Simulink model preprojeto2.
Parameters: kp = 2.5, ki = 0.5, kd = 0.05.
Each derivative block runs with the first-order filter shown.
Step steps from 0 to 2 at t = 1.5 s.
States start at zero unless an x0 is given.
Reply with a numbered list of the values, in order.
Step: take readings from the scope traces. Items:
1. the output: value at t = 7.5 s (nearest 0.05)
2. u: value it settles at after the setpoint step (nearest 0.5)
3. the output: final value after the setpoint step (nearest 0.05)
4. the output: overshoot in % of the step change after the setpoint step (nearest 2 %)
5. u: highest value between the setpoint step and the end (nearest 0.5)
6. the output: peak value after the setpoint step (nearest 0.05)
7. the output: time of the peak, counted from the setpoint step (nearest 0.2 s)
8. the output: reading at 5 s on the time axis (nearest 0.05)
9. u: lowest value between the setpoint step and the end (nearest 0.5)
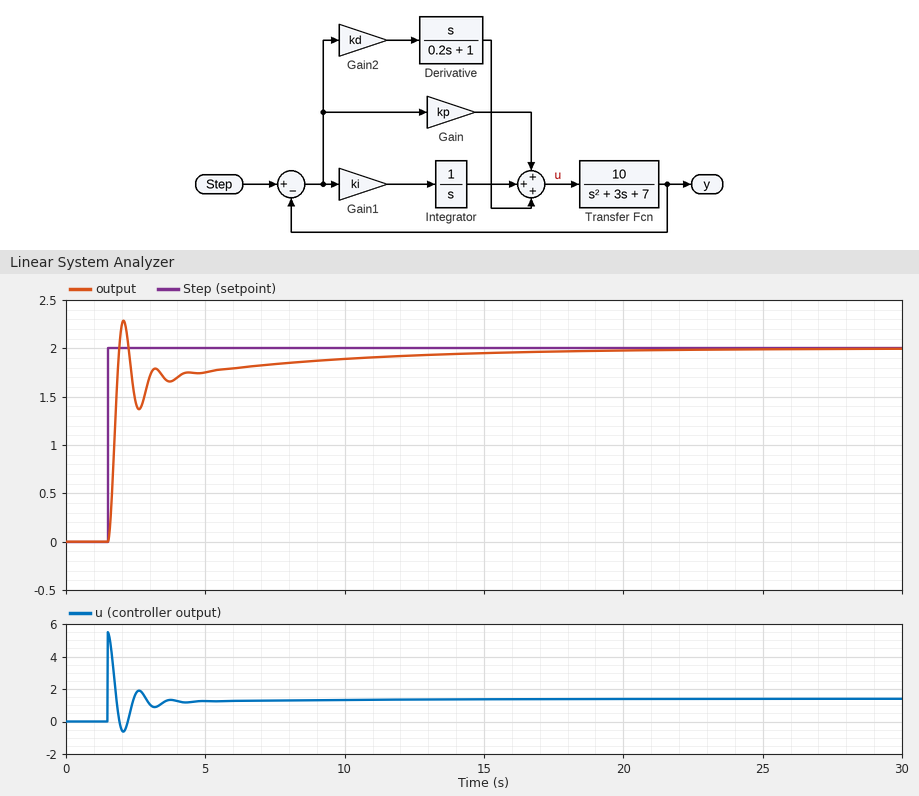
1. 1.85
2. 1.5
3. 2.00
4. 14 %
5. 5.5
6. 2.30
7. 0.6 s
8. 1.75
9. -0.5
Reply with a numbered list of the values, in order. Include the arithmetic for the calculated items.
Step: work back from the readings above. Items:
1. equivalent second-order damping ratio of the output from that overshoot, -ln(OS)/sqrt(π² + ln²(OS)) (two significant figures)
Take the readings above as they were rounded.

1. ln(0.14) = -1.966; 1.966 / sqrt(9.870 + 3.866) = 0.53
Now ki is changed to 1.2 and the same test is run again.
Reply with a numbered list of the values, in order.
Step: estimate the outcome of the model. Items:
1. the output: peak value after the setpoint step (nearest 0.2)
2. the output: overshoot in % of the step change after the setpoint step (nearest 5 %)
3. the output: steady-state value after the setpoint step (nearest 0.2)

1. 2.4
2. 20 %
3. 2.0
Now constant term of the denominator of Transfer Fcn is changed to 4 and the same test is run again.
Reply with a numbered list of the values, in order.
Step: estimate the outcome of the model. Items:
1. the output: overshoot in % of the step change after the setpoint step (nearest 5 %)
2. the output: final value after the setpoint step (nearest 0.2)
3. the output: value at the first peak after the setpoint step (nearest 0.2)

1. 25 %
2. 2.0
3. 2.4
